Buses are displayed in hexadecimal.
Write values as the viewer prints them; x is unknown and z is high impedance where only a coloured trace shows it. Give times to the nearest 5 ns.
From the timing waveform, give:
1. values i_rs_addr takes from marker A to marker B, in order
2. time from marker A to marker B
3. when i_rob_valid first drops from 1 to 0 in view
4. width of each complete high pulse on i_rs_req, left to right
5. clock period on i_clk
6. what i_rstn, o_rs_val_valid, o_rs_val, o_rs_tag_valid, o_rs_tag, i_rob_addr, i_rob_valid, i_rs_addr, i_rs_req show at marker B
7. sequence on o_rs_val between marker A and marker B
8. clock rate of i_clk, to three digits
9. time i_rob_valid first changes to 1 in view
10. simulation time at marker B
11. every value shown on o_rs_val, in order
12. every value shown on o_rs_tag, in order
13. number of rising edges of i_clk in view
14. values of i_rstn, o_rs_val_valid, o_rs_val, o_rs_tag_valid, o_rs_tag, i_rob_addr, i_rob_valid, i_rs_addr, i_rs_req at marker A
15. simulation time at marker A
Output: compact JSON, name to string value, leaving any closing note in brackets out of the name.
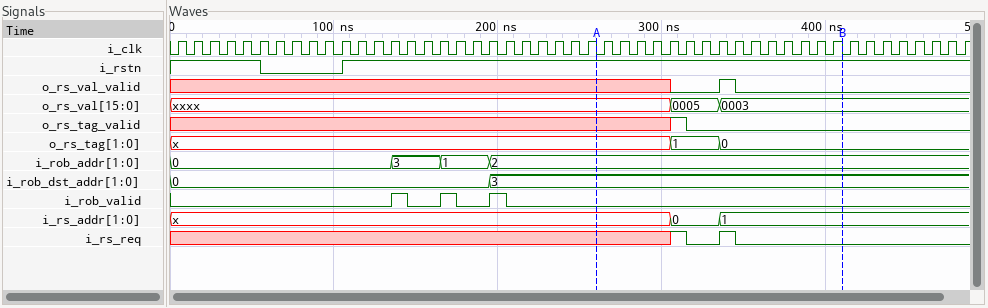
{"values i_rs_addr takes from marker A to marker B, in order": "x, 0, 1", "time from marker A to marker B": "150 ns", "when i_rob_valid first drops from 1 to 0 in view": "145 ns", "width of each complete high pulse on i_rs_req, left to right": "10 ns", "clock period on i_clk": "10 ns", "what i_rstn, o_rs_val_valid, o_rs_val, o_rs_tag_valid, o_rs_tag, i_rob_addr, i_rob_valid, i_rs_addr, i_rs_req show at marker B": "i_rstn=1, o_rs_val_valid=0, o_rs_val=0003, o_rs_tag_valid=0, o_rs_tag=0, i_rob_addr=2, i_rob_valid=0, i_rs_addr=1, i_rs_req=0", "sequence on o_rs_val between marker A and marker B": "xxxx, 0005, 0003", "clock rate of i_clk, to three digits": "100 MHz", "time i_rob_valid first changes to 1 in view": "135 ns", "simulation time at marker B": "410 ns", "every value shown on o_rs_val, in order": "xxxx, 0005, 0003", "every value shown on o_rs_tag, in order": "x, 1, 0", "number of rising edges of i_clk in view": "49", "values of i_rstn, o_rs_val_valid, o_rs_val, o_rs_tag_valid, o_rs_tag, i_rob_addr, i_rob_valid, i_rs_addr, i_rs_req at marker A": "i_rstn=1, o_rs_val_valid=x, o_rs_val=xxxx, o_rs_tag_valid=x, o_rs_tag=x, i_rob_addr=2, i_rob_valid=0, i_rs_addr=x, i_rs_req=x", "simulation time at marker A": "260 ns"}
